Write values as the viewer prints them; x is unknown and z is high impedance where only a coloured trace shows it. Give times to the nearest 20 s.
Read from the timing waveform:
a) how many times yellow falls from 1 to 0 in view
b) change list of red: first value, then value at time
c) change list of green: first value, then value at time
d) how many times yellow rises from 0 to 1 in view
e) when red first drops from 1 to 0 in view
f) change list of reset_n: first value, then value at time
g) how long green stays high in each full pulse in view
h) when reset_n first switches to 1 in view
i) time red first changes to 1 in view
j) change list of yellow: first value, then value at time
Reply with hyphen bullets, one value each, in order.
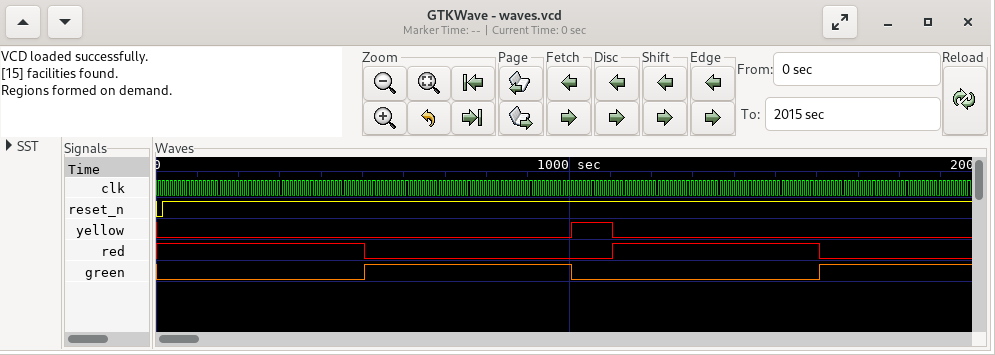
- 1
- 1, 0 at 500 s, 1 at 1100 s, 0 at 1600 s
- 0, 1 at 500 s, 0 at 1000 s, 1 at 1600 s
- 1
- 500 s
- 0, 1 at 20 s
- 500 s
- 20 s
- 1100 s
- 0, 1 at 1000 s, 0 at 1100 s
